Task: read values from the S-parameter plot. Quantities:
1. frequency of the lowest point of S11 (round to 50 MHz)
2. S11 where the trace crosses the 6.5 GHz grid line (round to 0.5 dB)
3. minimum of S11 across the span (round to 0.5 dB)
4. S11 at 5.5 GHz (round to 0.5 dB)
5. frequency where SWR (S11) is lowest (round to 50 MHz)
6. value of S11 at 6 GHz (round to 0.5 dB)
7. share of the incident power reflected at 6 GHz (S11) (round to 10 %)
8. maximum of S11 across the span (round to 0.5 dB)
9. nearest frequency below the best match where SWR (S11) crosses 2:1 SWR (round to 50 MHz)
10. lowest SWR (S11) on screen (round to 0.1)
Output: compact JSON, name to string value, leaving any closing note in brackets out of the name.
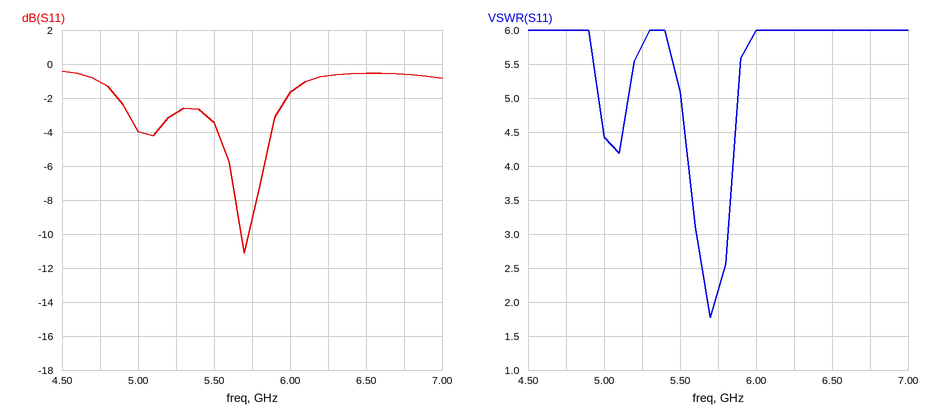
{"frequency of the lowest point of S11": "5.70 GHz", "S11 where the trace crosses the 6.5 GHz grid line": "-0.5 dB", "minimum of S11 across the span": "-11.0 dB", "S11 at 5.5 GHz": "-3.5 dB", "frequency where SWR (S11) is lowest": "5.70 GHz", "value of S11 at 6 GHz": "-1.5 dB", "share of the incident power reflected at 6 GHz (S11)": "70 %", "maximum of S11 across the span": "-0.5 dB", "nearest frequency below the best match where SWR (S11) crosses 2:1 SWR": "5.70 GHz", "lowest SWR (S11) on screen": "1.8"}
